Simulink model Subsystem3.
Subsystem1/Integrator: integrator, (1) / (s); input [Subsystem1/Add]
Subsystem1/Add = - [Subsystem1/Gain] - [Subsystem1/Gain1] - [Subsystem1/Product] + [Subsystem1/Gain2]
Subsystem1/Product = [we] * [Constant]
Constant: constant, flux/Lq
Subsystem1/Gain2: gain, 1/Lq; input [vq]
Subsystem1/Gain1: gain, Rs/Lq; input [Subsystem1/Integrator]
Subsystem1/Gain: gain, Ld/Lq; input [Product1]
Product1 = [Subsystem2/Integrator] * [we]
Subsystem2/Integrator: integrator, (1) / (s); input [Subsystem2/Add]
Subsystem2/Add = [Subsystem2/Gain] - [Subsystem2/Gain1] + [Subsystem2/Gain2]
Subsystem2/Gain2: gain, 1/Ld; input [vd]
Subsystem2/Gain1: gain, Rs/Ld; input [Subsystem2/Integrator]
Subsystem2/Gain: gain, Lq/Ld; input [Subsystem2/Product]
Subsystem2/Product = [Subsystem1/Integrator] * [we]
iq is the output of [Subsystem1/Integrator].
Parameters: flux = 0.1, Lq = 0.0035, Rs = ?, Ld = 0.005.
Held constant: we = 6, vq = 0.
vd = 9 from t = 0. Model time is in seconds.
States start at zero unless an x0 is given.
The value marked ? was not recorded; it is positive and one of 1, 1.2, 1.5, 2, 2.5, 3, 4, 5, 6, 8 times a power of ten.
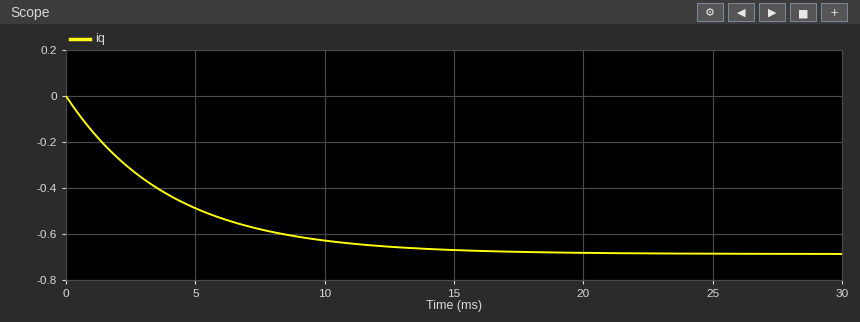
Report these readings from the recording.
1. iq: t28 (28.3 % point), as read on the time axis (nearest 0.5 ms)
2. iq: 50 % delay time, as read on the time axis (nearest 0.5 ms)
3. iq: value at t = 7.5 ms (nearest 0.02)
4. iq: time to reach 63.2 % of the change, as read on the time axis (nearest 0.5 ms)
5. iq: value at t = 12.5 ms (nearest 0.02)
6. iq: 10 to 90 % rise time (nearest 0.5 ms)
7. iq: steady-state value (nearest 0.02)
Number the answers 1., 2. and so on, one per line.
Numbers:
1. 1.5 ms
2. 3.0 ms
3. -0.58
4. 4.0 ms
5. -0.66
6. 9.0 ms
7. -0.68
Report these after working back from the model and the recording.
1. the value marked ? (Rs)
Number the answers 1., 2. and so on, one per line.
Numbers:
1. 1.2
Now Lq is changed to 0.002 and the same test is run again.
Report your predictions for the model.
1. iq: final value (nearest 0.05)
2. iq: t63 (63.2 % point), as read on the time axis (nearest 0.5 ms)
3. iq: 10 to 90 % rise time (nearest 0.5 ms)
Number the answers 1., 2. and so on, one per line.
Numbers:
1. -0.70
2. 2.5 ms
3. 6.5 ms
